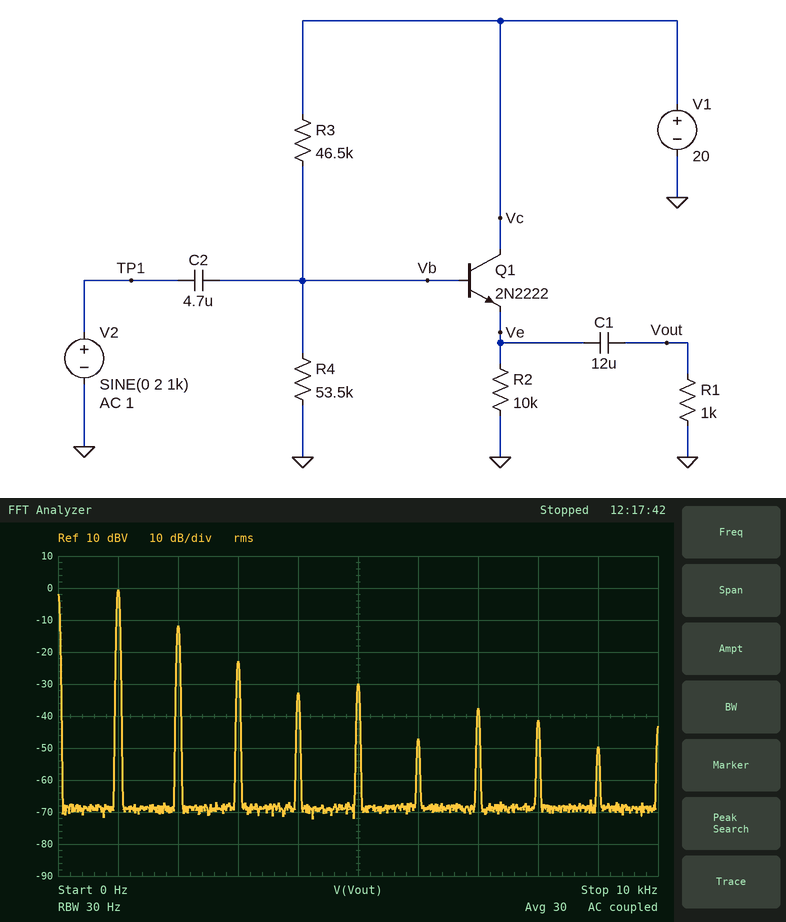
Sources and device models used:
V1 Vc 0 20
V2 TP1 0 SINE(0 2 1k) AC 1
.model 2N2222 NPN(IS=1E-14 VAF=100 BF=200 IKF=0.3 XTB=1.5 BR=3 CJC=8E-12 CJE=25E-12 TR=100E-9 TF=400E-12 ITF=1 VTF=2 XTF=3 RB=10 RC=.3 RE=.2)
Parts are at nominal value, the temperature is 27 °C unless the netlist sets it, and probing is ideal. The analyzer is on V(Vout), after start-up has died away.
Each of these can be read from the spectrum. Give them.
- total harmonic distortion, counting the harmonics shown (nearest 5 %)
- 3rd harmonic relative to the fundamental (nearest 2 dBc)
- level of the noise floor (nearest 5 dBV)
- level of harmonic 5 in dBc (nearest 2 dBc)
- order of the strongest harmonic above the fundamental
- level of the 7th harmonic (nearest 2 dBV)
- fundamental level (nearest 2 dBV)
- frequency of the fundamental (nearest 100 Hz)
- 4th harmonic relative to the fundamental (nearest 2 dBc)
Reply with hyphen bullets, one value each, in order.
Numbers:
- 30 %
- -22 dBc
- -70 dBV
- -30 dBc
- 2
- -38 dBV
- 0 dBV
- 1.0 kHz
- -32 dBc
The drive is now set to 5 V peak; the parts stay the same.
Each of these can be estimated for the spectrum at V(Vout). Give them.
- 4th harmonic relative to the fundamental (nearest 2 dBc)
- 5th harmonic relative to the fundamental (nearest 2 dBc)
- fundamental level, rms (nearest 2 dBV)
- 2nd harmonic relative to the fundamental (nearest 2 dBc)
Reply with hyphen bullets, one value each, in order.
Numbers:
- -22 dBc
- -24 dBc
- 2 dBV
- -6 dBc
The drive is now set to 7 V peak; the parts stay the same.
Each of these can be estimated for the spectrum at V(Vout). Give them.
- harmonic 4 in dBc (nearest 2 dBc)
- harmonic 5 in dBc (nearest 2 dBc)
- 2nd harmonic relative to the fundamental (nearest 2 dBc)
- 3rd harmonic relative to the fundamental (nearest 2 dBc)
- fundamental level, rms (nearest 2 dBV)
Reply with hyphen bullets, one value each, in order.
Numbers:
- -26 dBc
- -22 dBc
- -4 dBc
- -14 dBc
- 4 dBV
